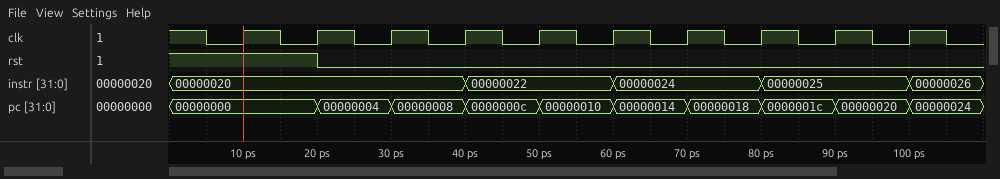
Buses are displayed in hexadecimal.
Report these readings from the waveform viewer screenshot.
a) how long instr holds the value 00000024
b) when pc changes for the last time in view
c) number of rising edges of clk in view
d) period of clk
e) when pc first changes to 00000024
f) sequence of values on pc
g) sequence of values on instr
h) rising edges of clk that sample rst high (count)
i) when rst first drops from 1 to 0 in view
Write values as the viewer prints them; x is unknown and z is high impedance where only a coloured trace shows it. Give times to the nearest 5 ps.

20 ps
100 ps
10
10 ps
100 ps
00000000, 00000004, 00000008, 0000000c, 00000010, 00000014, 00000018, 0000001c, 00000020, 00000024
00000020, 00000022, 00000024, 00000025, 00000026
2
20 ps
